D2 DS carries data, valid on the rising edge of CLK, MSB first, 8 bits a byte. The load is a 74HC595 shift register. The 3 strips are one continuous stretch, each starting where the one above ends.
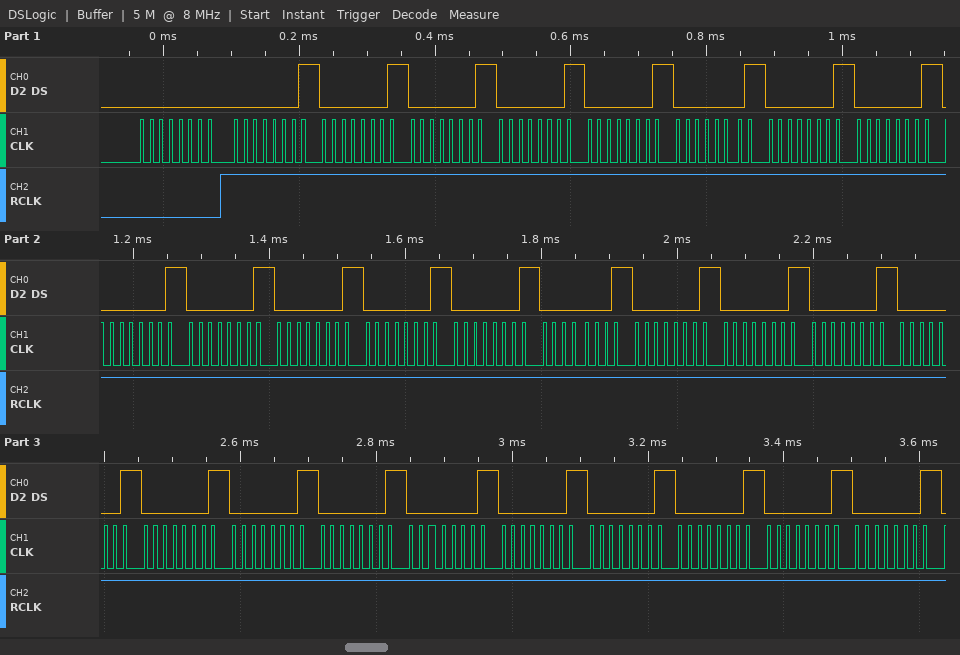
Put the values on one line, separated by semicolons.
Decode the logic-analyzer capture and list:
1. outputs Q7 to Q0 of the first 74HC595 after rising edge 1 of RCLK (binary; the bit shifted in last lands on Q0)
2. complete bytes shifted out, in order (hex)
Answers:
00000000; 00 01 01 01 01 01 01 01 01 01 01 01 01 01 01 01 01 01 01 01 01 01 01 01 01 01 01 01
